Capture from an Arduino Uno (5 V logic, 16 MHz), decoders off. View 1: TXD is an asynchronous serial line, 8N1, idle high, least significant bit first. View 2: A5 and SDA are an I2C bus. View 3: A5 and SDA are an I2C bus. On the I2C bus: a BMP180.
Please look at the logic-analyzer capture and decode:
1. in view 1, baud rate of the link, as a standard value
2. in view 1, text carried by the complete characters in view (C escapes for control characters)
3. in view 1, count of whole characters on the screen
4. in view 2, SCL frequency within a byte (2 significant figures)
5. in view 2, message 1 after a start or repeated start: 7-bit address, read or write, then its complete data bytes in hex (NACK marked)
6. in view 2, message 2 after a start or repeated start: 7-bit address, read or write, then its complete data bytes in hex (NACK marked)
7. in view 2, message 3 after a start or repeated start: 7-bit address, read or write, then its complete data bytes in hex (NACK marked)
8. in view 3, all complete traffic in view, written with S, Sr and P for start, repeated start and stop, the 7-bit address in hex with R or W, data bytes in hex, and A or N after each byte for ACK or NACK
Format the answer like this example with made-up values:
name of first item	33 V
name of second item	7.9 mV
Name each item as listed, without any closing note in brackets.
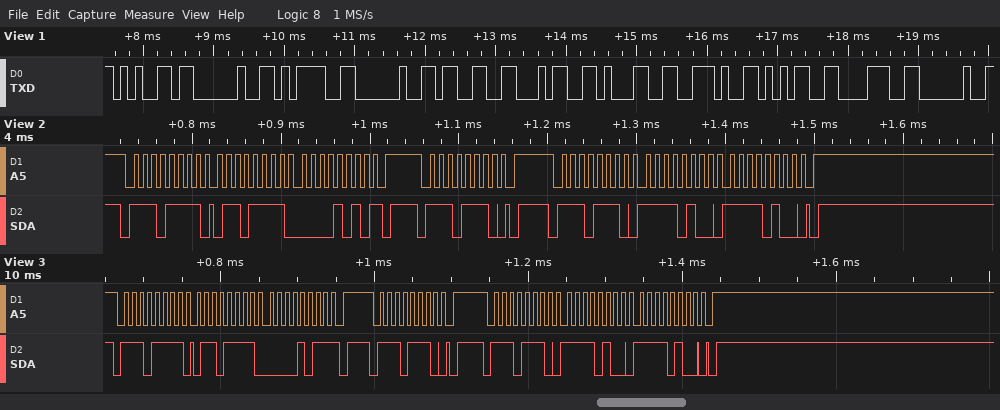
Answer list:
in view 1, baud rate of the link, as a standard value	9600 baud
in view 1, text carried by the complete characters in view	"e = 341.58 "
in view 1, count of whole characters on the screen	11
in view 2, SCL frequency within a byte	100 kHz
in view 2, message 1 after a start or repeated start: 7-bit address, read or write, then its complete data bytes in hex	0x77 read: 6F 0A NACK
in view 2, message 2 after a start or repeated start: 7-bit address, read or write, then its complete data bytes in hex	0x77 write
in view 2, message 3 after a start or repeated start: 7-bit address, read or write, then its complete data bytes in hex	0x77 write: F4 F4
in view 3, all complete traffic in view, written with S, Sr and P for start, repeated start and stop, the 7-bit address in hex with R or W, data bytes in hex, and A or N after each byte for ACK or NACK	S 77R A 6F A 0B N P S 77W A P S 77W A F4 A F4 A P
